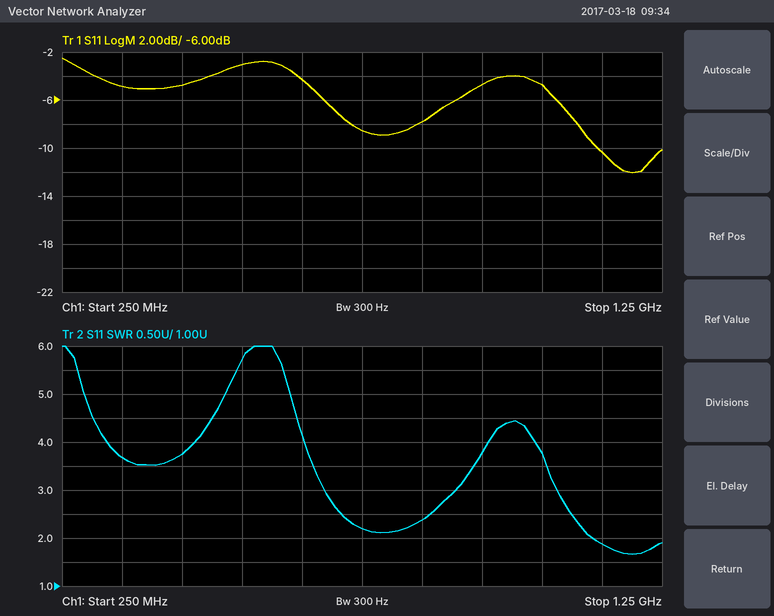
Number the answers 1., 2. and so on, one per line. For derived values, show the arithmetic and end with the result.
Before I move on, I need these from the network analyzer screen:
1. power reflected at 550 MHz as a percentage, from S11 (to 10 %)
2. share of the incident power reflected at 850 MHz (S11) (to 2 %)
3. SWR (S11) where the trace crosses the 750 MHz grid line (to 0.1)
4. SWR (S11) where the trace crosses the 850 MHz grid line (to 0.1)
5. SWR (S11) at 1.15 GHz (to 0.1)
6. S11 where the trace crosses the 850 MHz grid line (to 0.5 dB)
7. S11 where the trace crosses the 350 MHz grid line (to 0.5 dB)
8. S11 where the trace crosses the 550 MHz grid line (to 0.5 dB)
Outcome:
1. 10^(-3/10) ≈ 50 %
2. 10^(-8/10) ≈ 16 %
3. 2.2
4. 2.4
5. 1.9
6. -8.0 dB
7. -5.0 dB
8. -3.0 dB
